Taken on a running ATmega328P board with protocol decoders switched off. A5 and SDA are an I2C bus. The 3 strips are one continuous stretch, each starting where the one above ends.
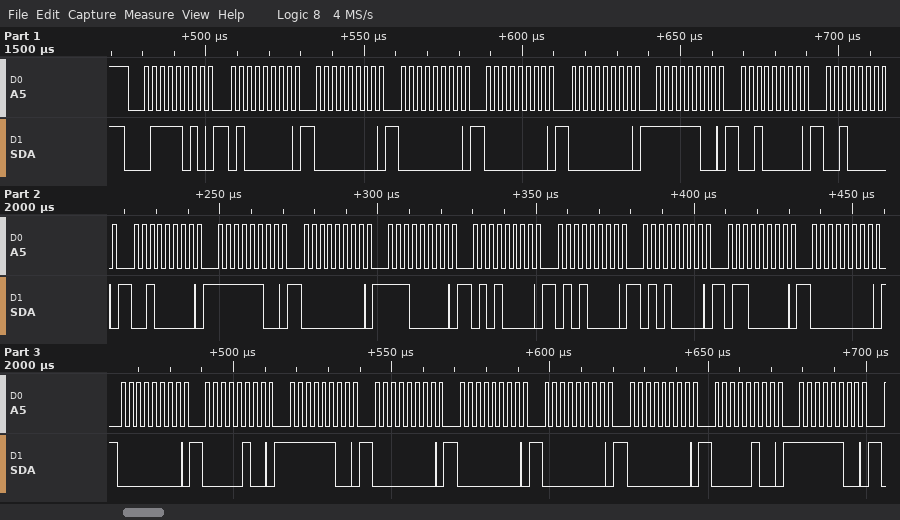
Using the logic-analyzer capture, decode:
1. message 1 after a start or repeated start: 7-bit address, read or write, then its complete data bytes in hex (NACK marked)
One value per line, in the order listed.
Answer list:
0x3D write: 40 00 00 00 00 FC 20 20 20 FC 00 E0 50 50 50 60 00 00 04 FC 00 00 00 00 04 FC
